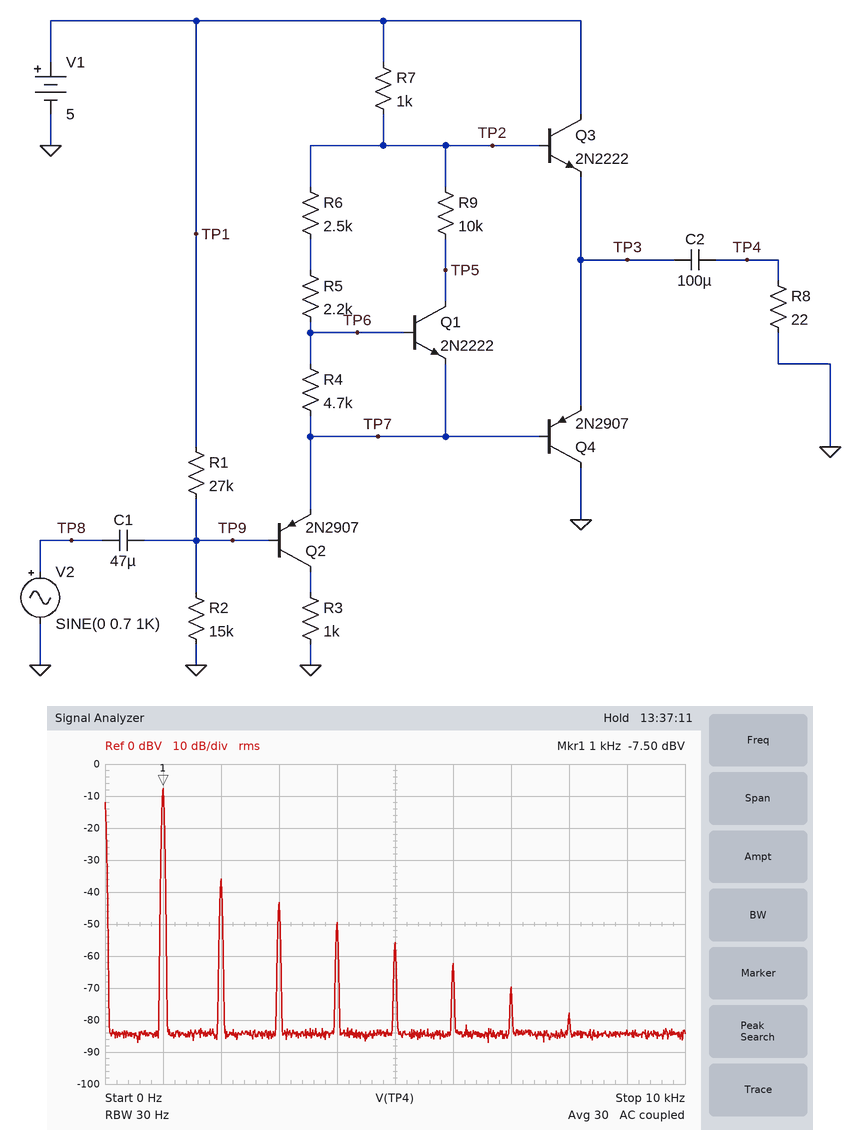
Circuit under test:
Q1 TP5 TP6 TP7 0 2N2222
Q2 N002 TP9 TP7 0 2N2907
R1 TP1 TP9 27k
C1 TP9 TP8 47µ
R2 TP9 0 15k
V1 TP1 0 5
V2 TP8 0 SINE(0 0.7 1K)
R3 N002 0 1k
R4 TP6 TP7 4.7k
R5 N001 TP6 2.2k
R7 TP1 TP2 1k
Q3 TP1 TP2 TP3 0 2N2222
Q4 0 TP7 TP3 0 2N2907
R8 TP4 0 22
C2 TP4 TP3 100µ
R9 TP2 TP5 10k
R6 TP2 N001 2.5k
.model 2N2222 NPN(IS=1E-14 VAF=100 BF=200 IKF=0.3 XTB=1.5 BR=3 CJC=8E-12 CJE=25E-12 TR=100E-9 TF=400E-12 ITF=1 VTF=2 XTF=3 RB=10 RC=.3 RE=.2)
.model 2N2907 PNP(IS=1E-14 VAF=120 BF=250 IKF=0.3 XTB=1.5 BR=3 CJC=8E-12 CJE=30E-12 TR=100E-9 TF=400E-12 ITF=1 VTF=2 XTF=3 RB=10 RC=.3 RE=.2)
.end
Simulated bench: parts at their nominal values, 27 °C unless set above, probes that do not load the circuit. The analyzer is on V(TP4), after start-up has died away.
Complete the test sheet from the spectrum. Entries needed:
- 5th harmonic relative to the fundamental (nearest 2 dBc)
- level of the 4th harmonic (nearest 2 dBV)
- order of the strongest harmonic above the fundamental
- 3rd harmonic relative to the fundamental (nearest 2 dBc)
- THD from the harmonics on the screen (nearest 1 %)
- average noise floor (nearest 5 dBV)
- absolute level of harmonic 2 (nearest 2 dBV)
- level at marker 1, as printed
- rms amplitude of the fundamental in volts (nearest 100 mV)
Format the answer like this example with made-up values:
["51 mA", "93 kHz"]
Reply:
["-48 dBc", "-50 dBV", "2", "-36 dBc", "4 %", "-85 dBV", "-36 dBV", "-7.50 dBV", "400 mV"]
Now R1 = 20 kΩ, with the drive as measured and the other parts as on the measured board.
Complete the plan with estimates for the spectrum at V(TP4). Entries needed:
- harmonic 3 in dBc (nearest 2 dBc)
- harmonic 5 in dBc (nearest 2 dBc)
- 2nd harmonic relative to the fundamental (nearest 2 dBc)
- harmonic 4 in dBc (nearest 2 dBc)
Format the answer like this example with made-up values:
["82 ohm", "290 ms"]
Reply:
["-26 dBc", "-40 dBc", "-18 dBc", "-44 dBc"]
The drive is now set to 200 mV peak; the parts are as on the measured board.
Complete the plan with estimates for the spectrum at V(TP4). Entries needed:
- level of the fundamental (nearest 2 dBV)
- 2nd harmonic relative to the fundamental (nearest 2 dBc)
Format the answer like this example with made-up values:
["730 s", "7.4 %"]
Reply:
["-18 dBV", "-46 dBc"]
